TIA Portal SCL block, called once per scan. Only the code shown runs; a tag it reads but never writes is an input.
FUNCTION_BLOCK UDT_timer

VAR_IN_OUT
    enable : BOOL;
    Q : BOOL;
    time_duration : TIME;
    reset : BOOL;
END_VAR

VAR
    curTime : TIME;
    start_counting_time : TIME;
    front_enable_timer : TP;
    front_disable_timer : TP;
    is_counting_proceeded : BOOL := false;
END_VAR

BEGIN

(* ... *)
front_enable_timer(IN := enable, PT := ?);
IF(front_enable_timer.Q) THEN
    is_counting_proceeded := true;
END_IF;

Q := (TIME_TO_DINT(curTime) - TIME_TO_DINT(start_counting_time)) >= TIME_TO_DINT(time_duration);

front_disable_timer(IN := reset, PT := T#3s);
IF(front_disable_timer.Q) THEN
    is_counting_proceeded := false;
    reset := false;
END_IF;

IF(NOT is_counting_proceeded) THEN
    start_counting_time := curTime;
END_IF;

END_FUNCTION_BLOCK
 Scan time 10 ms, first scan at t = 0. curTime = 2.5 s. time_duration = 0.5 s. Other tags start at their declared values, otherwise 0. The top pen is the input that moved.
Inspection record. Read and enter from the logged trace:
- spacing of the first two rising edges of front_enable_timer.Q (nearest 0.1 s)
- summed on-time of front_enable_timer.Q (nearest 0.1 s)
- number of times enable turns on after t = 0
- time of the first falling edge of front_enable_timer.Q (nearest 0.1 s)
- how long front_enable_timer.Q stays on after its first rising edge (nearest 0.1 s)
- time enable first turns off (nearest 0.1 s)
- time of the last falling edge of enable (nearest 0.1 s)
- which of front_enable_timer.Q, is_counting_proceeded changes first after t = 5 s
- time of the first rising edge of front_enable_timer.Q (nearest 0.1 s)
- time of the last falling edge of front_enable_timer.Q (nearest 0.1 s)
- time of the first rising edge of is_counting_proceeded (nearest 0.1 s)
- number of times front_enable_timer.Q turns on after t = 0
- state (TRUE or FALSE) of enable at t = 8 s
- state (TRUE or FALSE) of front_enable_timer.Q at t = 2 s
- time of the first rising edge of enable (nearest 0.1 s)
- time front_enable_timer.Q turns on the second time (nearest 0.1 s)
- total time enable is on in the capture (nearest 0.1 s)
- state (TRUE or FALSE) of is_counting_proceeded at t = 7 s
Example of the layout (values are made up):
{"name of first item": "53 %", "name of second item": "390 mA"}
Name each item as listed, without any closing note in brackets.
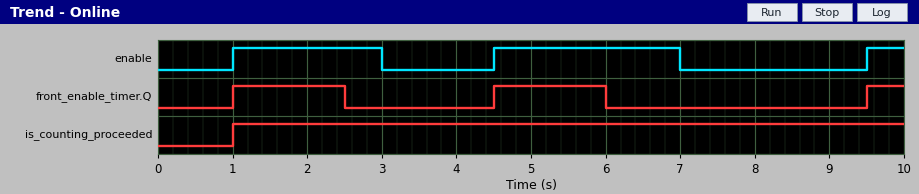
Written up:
{"spacing of the first two rising edges of front_enable_timer.Q": "3.5 s", "summed on-time of front_enable_timer.Q": "3.5 s", "number of times enable turns on after t = 0": "3", "time of the first falling edge of front_enable_timer.Q": "2.5 s", "how long front_enable_timer.Q stays on after its first rising edge": "1.5 s", "time enable first turns off": "3.0 s", "time of the last falling edge of enable": "7.0 s", "which of front_enable_timer.Q, is_counting_proceeded changes first after t = 5 s": "front_enable_timer.Q", "time of the first rising edge of front_enable_timer.Q": "1.0 s", "time of the last falling edge of front_enable_timer.Q": "6.0 s", "time of the first rising edge of is_counting_proceeded": "1.0 s", "number of times front_enable_timer.Q turns on after t = 0": "3", "state (TRUE or FALSE) of enable at t = 8 s": "FALSE", "state (TRUE or FALSE) of front_enable_timer.Q at t = 2 s": "TRUE", "time of the first rising edge of enable": "1.0 s", "time front_enable_timer.Q turns on the second time": "4.5 s", "total time enable is on in the capture": "5.0 s", "state (TRUE or FALSE) of is_counting_proceeded at t = 7 s": "TRUE"}
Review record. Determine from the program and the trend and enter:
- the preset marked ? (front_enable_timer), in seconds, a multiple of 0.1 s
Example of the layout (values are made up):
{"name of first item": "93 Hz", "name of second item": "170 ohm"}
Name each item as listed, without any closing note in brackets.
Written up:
{"the preset marked ? (front_enable_timer), in seconds, a multiple of 0.1 s": "1.5 s"}
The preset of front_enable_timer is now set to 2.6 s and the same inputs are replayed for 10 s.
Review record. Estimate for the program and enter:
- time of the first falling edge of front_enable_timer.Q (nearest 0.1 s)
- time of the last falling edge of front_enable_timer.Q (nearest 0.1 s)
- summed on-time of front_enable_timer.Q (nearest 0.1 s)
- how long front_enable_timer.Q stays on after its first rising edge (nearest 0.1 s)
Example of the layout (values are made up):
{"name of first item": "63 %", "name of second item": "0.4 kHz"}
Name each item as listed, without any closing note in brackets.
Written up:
{"time of the first falling edge of front_enable_timer.Q": "3.6 s", "time of the last falling edge of front_enable_timer.Q": "7.1 s", "summed on-time of front_enable_timer.Q": "5.7 s", "how long front_enable_timer.Q stays on after its first rising edge": "2.6 s"}
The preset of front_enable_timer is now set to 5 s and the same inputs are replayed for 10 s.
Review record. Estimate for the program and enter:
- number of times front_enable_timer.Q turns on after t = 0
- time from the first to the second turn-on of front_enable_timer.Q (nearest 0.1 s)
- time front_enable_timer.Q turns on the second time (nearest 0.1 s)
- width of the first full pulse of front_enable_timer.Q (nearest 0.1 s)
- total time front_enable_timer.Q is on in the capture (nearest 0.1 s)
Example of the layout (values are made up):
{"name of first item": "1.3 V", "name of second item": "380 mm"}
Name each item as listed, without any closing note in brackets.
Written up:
{"number of times front_enable_timer.Q turns on after t = 0": "2", "time from the first to the second turn-on of front_enable_timer.Q": "8.5 s", "time front_enable_timer.Q turns on the second time": "9.5 s", "width of the first full pulse of front_enable_timer.Q": "5.0 s", "total time front_enable_timer.Q is on in the capture": "5.5 s"}
